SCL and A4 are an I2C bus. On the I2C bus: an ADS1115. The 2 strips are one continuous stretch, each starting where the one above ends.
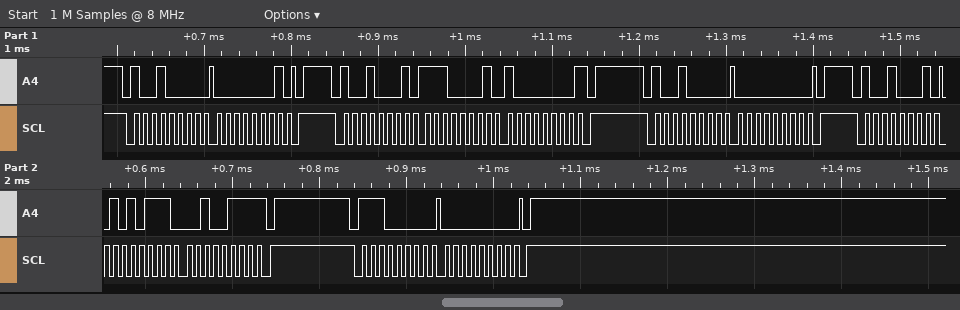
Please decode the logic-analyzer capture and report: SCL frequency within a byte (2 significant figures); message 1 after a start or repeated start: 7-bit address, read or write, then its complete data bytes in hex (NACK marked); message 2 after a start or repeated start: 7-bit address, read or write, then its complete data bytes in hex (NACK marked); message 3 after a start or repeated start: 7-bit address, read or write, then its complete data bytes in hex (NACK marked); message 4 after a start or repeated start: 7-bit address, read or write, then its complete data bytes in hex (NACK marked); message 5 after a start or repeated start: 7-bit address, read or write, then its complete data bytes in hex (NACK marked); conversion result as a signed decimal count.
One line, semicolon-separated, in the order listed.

100 kHz; 0x48 write: 01; 0x48 read: E1 80 NACK; 0x48 write: 00; 0x48 read: 57 27 NACK; 0x70 write: 00; 22311
